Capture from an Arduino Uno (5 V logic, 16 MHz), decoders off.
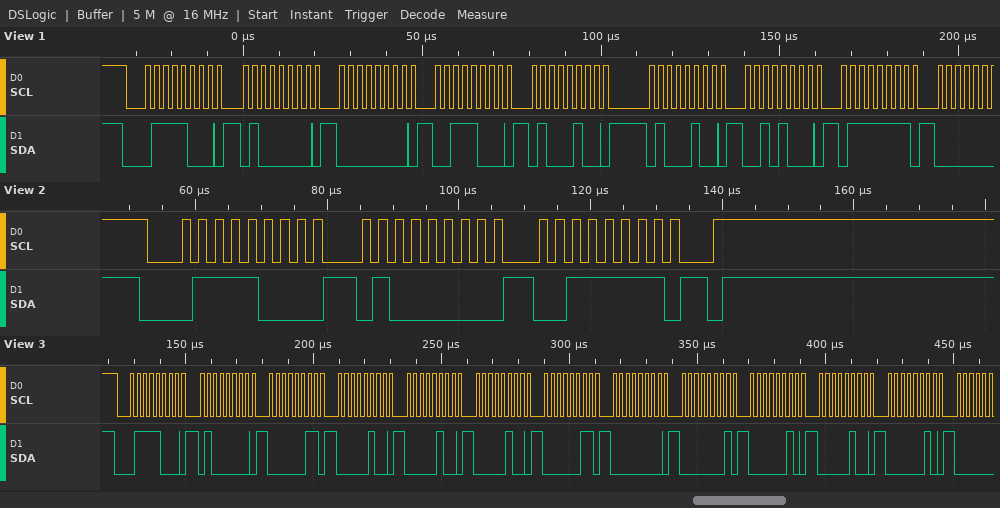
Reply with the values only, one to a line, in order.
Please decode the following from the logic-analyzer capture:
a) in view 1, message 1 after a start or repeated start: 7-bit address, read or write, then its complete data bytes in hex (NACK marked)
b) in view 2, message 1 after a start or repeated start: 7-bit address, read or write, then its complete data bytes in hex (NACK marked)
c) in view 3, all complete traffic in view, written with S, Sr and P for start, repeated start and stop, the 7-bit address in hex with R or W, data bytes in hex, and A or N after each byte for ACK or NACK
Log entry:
0x3C write: 40 00 38 44 44 28 7F
0x3C write: 40 3F
S 3CW A 40 A 03 A 04 A 04 A 04 A 03 A 00 A 01 A 02 A 04 A 02 A
